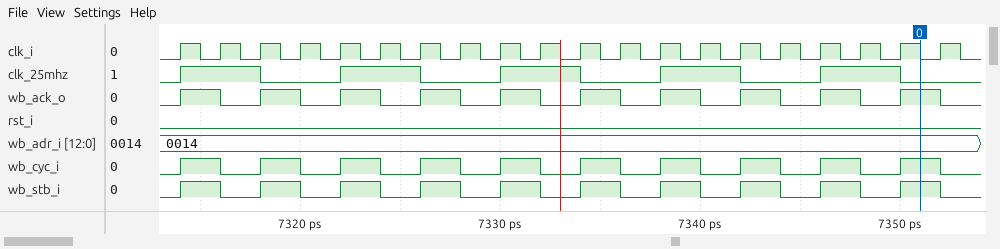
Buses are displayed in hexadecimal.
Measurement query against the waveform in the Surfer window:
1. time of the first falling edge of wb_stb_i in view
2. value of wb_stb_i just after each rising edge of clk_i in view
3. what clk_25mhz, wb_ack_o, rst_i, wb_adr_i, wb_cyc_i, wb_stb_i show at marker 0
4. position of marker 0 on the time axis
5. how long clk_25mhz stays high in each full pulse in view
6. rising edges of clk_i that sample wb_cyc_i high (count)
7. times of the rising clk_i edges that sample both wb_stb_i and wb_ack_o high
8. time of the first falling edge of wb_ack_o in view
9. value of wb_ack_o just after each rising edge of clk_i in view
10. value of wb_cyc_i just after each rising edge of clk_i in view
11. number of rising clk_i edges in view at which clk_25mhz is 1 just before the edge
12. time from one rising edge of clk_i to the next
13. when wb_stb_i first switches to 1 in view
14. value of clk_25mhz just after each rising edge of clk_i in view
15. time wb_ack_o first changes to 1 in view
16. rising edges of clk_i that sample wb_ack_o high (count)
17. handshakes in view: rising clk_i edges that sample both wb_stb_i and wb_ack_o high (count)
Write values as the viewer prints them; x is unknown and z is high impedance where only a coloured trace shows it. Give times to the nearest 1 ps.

7316 ps
1 0 1 0 1 0 1 0 1 0 1 0 1 0 1 0 1 0 1 0
clk_25mhz=0, wb_ack_o=1, rst_i=0, wb_adr_i=0014, wb_cyc_i=1, wb_stb_i=1
7351 ps
4 ps, 4 ps, 4 ps, 4 ps, 4 ps
10
7316 ps, 7320 ps, 7324 ps, 7328 ps, 7332 ps, 7336 ps, 7340 ps, 7344 ps, 7348 ps, 7352 ps
7316 ps
1 0 1 0 1 0 1 0 1 0 1 0 1 0 1 0 1 0 1 0
1 0 1 0 1 0 1 0 1 0 1 0 1 0 1 0 1 0 1 0
10
2 ps
7314 ps
1 1 0 0 1 1 0 0 1 1 0 0 1 1 0 0 1 1 0 0
7314 ps
10
10
